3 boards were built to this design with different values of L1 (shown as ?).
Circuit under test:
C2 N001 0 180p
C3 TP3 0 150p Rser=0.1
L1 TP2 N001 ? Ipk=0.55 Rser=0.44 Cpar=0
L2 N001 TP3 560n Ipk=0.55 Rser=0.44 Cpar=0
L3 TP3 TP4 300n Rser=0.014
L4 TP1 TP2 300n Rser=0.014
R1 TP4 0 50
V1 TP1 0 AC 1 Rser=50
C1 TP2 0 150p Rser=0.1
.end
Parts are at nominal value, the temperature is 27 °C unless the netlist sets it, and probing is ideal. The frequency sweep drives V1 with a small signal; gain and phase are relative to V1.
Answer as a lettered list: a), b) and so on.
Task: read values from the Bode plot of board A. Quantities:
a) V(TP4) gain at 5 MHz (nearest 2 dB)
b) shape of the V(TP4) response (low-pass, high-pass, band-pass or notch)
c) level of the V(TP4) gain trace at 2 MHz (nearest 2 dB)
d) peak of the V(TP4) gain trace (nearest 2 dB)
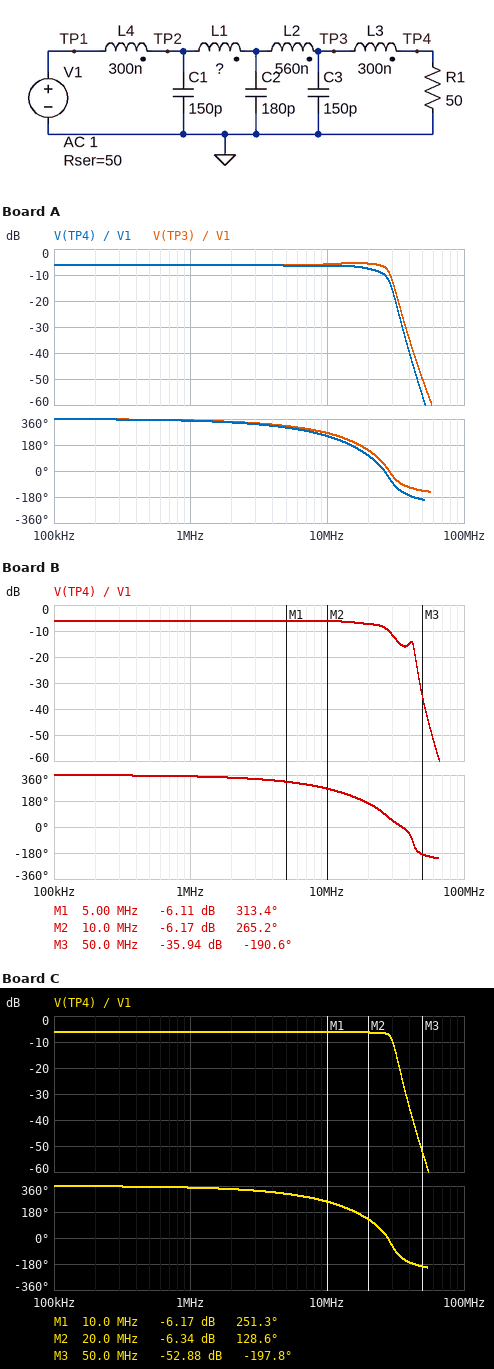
a) -6 dB
b) low-pass
c) -6 dB
d) -6 dB
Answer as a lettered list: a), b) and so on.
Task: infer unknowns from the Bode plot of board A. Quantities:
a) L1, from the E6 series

a) 1 µH
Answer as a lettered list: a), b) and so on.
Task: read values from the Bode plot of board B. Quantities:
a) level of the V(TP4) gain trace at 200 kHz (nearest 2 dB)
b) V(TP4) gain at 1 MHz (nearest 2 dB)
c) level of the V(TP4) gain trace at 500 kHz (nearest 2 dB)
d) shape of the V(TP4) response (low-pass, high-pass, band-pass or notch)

a) -6 dB
b) -6 dB
c) -6 dB
d) low-pass
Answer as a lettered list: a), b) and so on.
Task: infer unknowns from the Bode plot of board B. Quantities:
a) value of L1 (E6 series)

a) 220 nH
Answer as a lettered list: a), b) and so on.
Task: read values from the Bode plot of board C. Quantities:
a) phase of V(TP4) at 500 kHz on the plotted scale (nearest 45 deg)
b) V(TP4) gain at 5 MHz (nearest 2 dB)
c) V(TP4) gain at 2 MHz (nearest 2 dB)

a) 360 deg
b) -6 dB
c) -6 dB
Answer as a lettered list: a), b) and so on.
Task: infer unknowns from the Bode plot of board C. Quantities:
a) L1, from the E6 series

a) 680 nH
